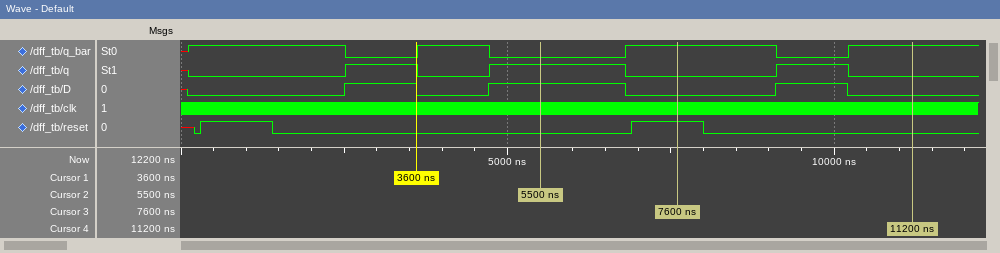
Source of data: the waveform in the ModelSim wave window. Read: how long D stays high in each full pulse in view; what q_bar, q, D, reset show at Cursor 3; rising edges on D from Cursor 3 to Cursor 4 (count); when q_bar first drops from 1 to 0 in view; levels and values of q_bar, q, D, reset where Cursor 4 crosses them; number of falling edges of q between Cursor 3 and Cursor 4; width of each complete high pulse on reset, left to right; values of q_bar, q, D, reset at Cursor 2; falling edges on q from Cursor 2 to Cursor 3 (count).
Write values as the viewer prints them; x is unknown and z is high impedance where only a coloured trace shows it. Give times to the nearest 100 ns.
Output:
1100 ns, 2100 ns, 1100 ns
q_bar=1, q=0, D=0, reset=1
1
2500 ns
q_bar=1, q=0, D=0, reset=0
1
1100 ns, 1100 ns
q_bar=0, q=1, D=1, reset=0
1
